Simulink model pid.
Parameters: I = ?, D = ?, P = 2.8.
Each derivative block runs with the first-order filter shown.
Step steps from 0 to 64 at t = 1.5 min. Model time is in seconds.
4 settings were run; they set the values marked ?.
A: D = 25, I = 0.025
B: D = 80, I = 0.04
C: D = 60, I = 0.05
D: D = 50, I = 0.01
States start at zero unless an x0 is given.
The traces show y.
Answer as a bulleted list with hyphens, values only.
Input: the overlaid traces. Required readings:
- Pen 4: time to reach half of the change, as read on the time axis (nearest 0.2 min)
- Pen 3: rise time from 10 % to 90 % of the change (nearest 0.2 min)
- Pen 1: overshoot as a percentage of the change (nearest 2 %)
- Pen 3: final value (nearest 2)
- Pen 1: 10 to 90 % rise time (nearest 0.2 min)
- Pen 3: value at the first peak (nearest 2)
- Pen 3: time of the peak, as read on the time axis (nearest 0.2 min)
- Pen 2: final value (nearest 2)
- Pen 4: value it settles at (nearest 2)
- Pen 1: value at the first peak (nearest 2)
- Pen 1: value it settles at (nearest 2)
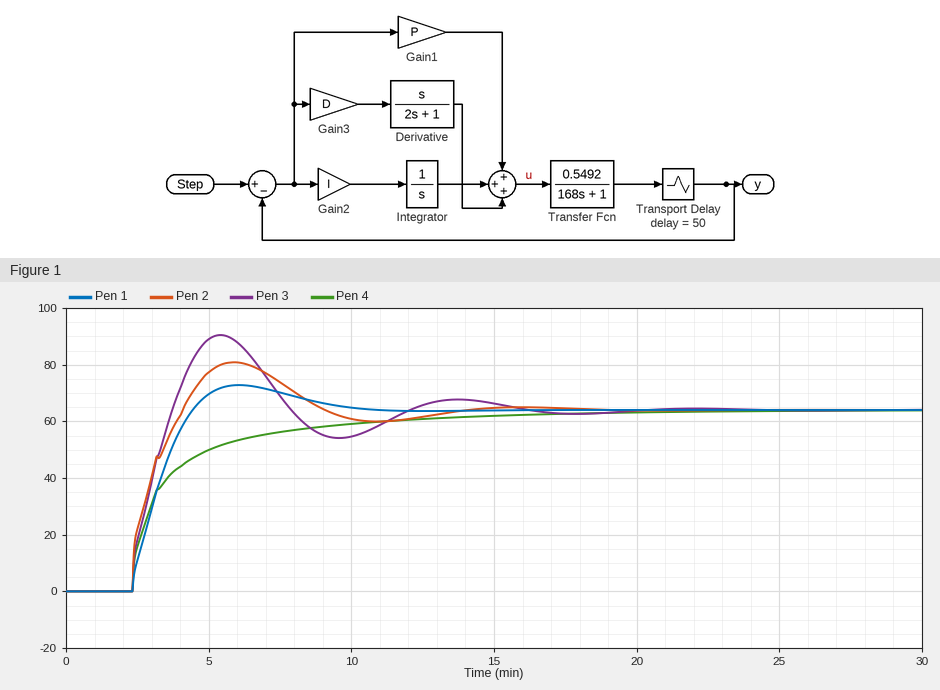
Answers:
- 3.0 min
- 1.2 min
- 14 %
- 64
- 1.6 min
- 90
- 5.4 min
- 64
- 64
- 72
- 64
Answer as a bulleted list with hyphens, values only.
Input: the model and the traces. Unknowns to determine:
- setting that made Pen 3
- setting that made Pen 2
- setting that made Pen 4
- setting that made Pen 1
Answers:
- C
- B
- D
- A
